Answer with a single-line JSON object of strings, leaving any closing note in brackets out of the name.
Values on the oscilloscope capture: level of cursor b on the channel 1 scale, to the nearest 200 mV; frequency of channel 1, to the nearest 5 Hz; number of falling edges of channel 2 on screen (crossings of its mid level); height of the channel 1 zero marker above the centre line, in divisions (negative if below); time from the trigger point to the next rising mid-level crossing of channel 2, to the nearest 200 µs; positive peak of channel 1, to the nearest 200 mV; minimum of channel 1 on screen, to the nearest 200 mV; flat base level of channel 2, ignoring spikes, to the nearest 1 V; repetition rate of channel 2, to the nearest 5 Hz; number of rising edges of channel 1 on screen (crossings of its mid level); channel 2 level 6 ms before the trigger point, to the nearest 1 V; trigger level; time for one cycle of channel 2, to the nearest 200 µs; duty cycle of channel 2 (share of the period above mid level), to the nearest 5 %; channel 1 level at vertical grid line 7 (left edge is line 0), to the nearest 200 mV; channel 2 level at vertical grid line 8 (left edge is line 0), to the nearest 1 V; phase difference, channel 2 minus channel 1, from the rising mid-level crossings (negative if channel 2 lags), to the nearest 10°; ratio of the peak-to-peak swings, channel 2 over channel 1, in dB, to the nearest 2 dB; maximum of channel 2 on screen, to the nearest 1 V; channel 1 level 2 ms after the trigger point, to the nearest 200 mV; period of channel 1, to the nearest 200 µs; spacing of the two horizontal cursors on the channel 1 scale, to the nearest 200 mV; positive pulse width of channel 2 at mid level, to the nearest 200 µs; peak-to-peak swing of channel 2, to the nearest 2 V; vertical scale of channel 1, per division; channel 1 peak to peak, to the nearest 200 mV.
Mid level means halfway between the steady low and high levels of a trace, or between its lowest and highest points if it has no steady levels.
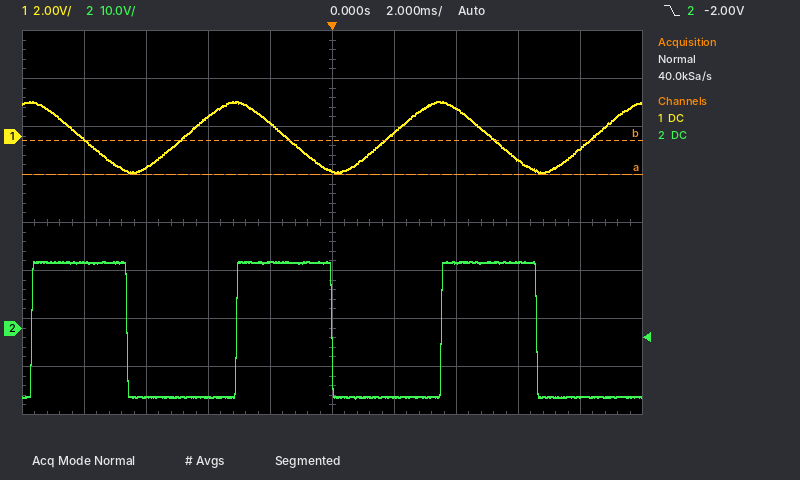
{"level of cursor b on the channel 1 scale, to the nearest 200 mV": "-200 mV", "frequency of channel 1, to the nearest 5 Hz": "150 Hz", "number of falling edges of channel 2 on screen": "3", "height of the channel 1 zero marker above the centre line, in divisions": "+1.8 div", "time from the trigger point to the next rising mid-level crossing of channel 2, to the nearest 200 µs": "3.6 ms", "positive peak of channel 1, to the nearest 200 mV": "1.4 V", "minimum of channel 1 on screen, to the nearest 200 mV": "-1.6 V", "flat base level of channel 2, ignoring spikes, to the nearest 1 V": "-14 V", "repetition rate of channel 2, to the nearest 5 Hz": "150 Hz", "number of rising edges of channel 1 on screen": "3", "channel 2 level 6 ms before the trigger point, to the nearest 1 V": "-14 V", "trigger level": "-2.00 V", "time for one cycle of channel 2, to the nearest 200 µs": "6.6 ms", "duty cycle of channel 2 (share of the period above mid level), to the nearest 5 %": "45 %", "channel 1 level at vertical grid line 7 (left edge is line 0), to the nearest 200 mV": "1.2 V", "channel 2 level at vertical grid line 8 (left edge is line 0), to the nearest 1 V": "14 V", "phase difference, channel 2 minus channel 1, from the rising mid-level crossings (negative if channel 2 lags), to the nearest 10°": "-90°", "ratio of the peak-to-peak swings, channel 2 over channel 1, in dB, to the nearest 2 dB": "20 dB", "maximum of channel 2 on screen, to the nearest 1 V": "14 V", "channel 1 level 2 ms after the trigger point, to the nearest 200 mV": "200 mV", "period of channel 1, to the nearest 200 µs": "6.6 ms", "spacing of the two horizontal cursors on the channel 1 scale, to the nearest 200 mV": "1.4 V", "positive pulse width of channel 2 at mid level, to the nearest 200 µs": "3.0 ms", "peak-to-peak swing of channel 2, to the nearest 2 V": "28 V", "vertical scale of channel 1, per division": "2 V", "channel 1 peak to peak, to the nearest 200 mV": "3.0 V"}
